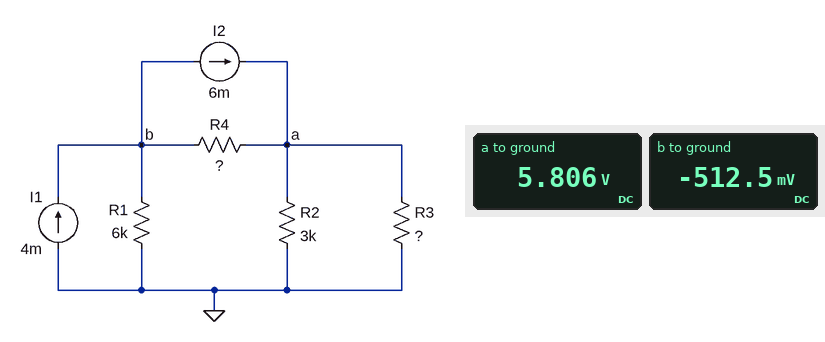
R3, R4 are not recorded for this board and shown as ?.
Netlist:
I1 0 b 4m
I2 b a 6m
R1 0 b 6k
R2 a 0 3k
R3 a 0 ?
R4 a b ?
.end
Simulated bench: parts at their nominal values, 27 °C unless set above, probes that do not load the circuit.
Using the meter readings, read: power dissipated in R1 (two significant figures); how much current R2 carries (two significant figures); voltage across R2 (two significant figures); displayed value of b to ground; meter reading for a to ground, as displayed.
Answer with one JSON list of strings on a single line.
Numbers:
["44 µW", "1.9 mA", "5.8 V", "-512.5 mV", "5.806 V"]
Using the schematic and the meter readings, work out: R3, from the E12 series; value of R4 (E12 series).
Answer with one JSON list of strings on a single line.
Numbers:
["2.7 kΩ", "3.3 kΩ"]
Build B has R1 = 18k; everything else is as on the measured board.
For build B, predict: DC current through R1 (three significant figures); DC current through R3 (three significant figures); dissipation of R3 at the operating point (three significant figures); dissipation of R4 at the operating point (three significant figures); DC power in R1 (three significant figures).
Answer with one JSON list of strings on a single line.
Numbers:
["40.3 µA", "2.13 mA", "12.2 mW", "12.7 mW", "29.2 µW"]
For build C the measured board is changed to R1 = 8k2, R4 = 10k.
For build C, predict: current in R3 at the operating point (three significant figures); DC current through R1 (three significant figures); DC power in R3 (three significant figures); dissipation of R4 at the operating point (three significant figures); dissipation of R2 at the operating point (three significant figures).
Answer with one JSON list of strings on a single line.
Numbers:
["2.49 mA", "730 µA", "16.7 mW", "16.1 mW", "15.1 mW"]
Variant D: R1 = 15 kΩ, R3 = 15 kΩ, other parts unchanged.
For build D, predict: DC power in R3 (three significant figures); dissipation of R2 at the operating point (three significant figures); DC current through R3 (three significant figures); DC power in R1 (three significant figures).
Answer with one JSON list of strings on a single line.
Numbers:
["6.13 mW", "30.7 mW", "639 µA", "401 µW"]
